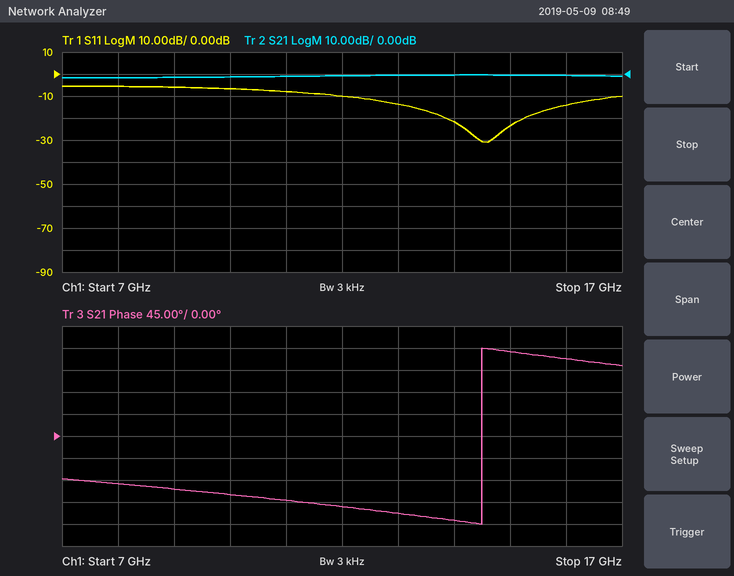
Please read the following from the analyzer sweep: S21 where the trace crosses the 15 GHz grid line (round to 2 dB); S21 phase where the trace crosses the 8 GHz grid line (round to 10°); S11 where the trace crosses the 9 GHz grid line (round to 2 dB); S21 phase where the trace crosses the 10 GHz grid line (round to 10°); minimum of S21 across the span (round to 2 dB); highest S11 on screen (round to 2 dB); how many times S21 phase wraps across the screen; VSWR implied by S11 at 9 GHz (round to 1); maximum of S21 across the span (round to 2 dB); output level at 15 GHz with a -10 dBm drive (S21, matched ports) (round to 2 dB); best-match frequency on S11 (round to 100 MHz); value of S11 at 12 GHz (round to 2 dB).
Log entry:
0 dB
-100°
-6 dB
-120°
-2 dB
-6 dB
1
3
0 dB
-10 dBm
14.6 GHz
-10 dB
